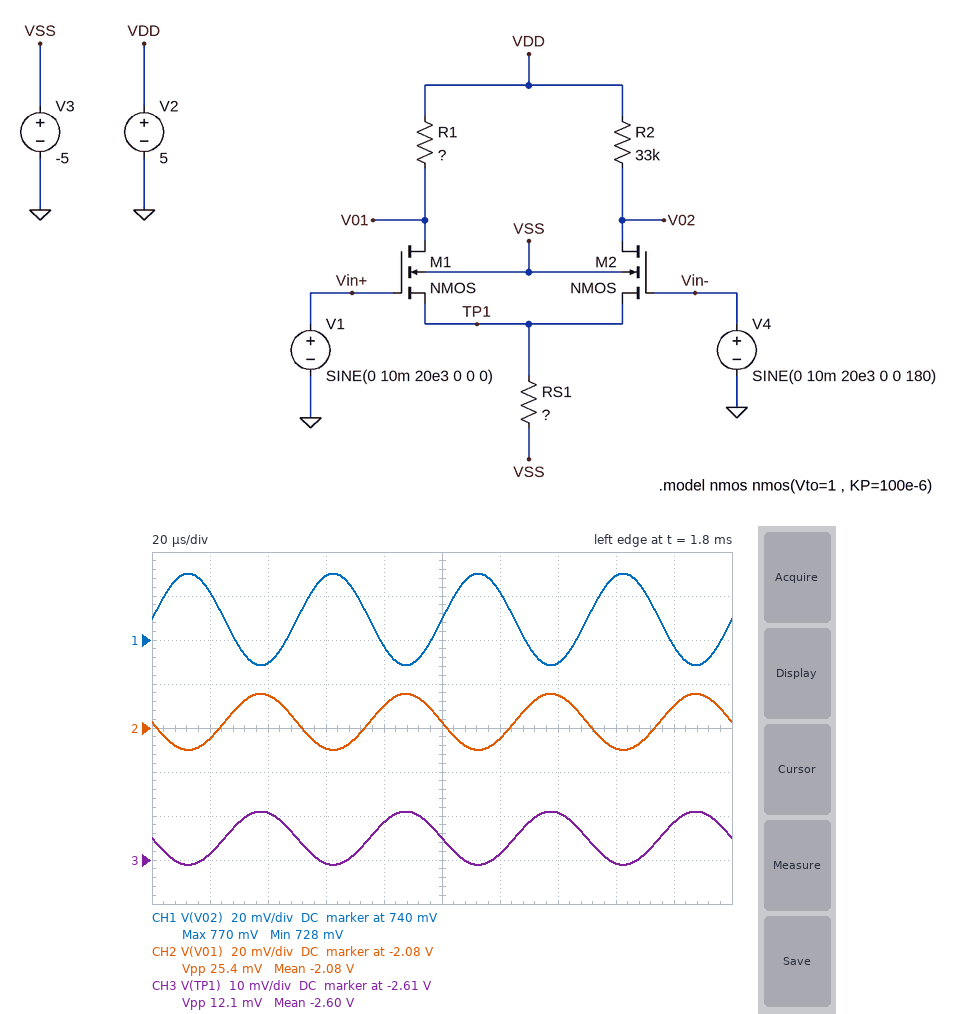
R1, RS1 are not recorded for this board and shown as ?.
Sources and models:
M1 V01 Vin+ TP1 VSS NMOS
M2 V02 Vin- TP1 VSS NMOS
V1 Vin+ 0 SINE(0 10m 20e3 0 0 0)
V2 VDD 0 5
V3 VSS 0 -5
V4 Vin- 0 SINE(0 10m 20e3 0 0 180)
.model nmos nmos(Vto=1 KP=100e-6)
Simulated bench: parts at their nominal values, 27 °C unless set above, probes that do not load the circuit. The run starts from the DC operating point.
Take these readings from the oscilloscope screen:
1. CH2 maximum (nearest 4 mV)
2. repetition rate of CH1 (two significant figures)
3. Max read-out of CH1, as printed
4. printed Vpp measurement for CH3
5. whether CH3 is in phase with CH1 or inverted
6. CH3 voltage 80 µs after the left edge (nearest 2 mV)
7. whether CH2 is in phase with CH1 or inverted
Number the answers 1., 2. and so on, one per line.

1. -2.064 V
2. 20 kHz
3. 770 mV
4. 12.1 mV
5. inverted
6. -2.602 V
7. inverted
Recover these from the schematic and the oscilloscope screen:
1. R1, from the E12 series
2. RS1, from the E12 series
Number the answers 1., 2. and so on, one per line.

1. 100 kΩ
2. 12 kΩ
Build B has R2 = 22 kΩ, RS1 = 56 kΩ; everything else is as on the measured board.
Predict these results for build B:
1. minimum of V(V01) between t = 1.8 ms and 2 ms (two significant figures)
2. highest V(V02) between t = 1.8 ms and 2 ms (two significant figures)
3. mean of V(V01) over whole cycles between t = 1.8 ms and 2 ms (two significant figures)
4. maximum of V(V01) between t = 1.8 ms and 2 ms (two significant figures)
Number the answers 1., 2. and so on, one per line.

1. 2.0 V
2. 4.4 V
3. 2.1 V
4. 2.2 V
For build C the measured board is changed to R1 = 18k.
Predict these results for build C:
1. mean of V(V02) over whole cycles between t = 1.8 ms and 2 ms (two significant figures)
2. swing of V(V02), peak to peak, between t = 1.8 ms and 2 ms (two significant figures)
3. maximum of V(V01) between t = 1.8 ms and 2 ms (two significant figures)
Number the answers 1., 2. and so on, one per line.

1. 1.5 V
2. 96 mV
3. 3.1 V
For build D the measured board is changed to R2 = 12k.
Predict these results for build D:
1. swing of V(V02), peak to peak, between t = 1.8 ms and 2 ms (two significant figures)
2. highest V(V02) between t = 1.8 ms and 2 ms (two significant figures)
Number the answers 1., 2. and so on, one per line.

1. 15 mV
2. 3.5 V
